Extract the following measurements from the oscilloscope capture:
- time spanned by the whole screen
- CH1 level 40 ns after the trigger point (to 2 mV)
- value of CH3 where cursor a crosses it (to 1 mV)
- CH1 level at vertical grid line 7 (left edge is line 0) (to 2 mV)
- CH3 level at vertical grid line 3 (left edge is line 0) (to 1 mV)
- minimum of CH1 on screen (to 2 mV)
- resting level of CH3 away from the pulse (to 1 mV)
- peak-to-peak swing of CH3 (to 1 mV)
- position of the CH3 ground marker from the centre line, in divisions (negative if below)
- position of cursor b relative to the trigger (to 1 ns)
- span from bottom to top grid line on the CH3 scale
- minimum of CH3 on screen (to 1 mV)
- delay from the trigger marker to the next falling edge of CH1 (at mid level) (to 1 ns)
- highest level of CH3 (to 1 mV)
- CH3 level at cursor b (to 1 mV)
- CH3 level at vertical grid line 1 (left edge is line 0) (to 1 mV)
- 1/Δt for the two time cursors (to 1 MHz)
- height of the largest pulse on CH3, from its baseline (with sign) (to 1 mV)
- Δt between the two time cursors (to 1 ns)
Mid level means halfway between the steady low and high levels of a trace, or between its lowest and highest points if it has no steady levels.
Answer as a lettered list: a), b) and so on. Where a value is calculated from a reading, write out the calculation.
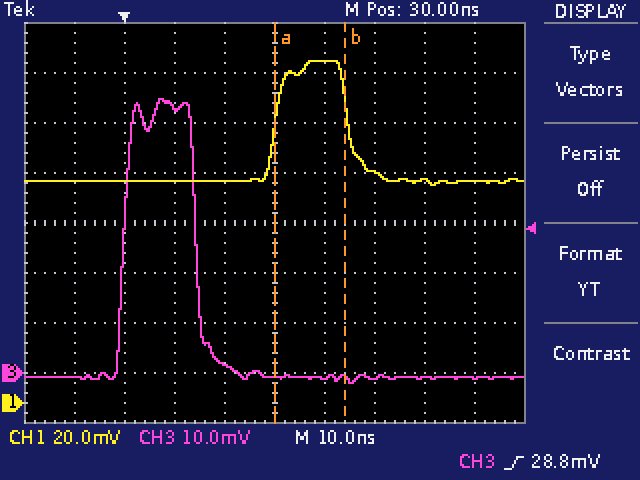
a) 100 ns
b) 136 mV
c) -1 mV
d) 92 mV
e) 53 mV
f) 88 mV
g) -1 mV
h) 55 mV − (-2 mV) = 57 mV
i) -3.0 div
j) +44 ns
k) 80 mV
l) -2 mV
m) 45 ns
n) 55 mV
o) -1 mV
p) -1 mV
q) 1 / 14 ns ≈ 71 MHz
r) 55 mV − (-1 mV) = +56 mV
s) 14 ns
